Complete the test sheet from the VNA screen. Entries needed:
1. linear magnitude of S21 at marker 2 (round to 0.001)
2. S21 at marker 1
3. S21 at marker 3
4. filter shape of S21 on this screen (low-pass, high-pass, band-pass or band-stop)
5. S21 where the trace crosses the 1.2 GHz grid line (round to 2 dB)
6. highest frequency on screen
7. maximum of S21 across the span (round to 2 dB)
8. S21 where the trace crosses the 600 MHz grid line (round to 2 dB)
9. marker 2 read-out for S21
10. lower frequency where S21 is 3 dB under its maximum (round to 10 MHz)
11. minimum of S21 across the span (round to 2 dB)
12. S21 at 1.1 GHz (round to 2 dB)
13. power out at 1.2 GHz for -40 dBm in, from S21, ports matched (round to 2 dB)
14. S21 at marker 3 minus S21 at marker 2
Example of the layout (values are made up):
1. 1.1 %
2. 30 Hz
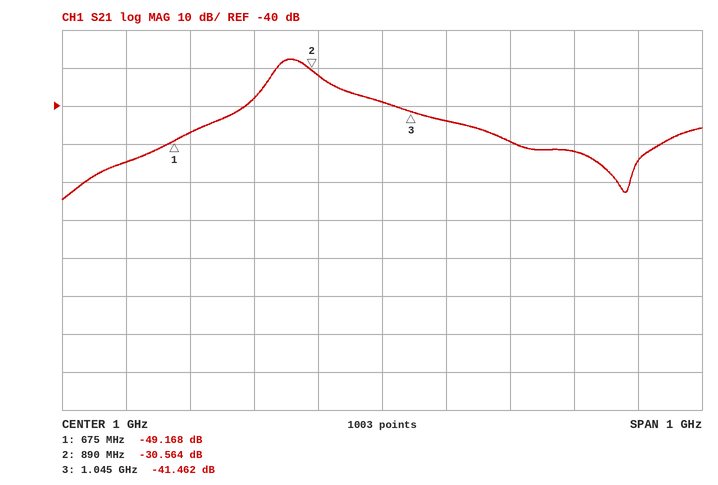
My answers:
1. 0.030
2. -49.168 dB
3. -41.462 dB
4. band-pass
5. -50 dB
6. 1.5 GHz
7. -28 dB
8. -54 dB
9. -30.564 dB
10. 830 MHz
11. -64 dB
12. -44 dB
13. -90 dBm
14. -10.898 dB
